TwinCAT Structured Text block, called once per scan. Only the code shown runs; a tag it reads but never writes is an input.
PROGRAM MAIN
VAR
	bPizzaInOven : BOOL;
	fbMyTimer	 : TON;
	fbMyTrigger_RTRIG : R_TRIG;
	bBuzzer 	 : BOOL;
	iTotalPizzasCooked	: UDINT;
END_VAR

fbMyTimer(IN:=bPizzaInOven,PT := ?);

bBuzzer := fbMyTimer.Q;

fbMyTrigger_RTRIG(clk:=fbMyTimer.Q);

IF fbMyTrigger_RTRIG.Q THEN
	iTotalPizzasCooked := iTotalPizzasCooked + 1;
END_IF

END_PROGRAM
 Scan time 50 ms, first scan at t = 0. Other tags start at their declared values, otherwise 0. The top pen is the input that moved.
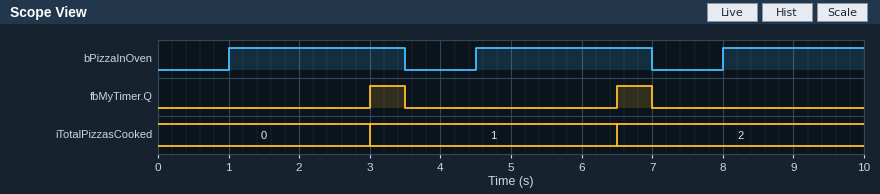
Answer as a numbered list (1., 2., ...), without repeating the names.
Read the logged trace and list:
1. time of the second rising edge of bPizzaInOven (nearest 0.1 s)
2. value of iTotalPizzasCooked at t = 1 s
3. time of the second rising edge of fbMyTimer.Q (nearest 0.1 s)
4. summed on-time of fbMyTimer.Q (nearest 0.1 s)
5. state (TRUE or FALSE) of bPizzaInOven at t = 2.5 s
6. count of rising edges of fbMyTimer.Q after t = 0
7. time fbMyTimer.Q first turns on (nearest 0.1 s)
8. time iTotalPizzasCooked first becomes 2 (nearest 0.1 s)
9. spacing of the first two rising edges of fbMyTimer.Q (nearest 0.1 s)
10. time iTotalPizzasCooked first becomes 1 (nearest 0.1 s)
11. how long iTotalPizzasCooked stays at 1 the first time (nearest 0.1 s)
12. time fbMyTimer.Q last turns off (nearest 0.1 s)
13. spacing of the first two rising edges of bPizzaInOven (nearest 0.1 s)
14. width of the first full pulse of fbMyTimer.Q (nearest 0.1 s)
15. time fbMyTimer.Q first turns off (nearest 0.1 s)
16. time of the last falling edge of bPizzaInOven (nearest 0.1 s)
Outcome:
1. 4.5 s
2. 0
3. 6.5 s
4. 1.0 s
5. TRUE
6. 2
7. 3.0 s
8. 6.5 s
9. 3.5 s
10. 3.0 s
11. 3.5 s
12. 7.0 s
13. 3.5 s
14. 0.5 s
15. 3.5 s
16. 7.0 s
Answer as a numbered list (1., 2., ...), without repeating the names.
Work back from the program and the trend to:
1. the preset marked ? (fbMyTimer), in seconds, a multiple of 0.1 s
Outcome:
1. 2.0 s
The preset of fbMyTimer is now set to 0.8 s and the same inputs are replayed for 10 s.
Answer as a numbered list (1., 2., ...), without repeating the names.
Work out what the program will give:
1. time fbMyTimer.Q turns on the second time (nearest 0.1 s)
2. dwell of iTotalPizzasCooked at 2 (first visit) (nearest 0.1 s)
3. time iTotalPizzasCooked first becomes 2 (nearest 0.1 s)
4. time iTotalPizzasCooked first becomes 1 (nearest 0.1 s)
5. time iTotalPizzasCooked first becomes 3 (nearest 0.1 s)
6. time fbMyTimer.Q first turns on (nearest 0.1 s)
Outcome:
1. 5.3 s
2. 3.5 s
3. 5.3 s
4. 1.8 s
5. 8.8 s
6. 1.8 s
